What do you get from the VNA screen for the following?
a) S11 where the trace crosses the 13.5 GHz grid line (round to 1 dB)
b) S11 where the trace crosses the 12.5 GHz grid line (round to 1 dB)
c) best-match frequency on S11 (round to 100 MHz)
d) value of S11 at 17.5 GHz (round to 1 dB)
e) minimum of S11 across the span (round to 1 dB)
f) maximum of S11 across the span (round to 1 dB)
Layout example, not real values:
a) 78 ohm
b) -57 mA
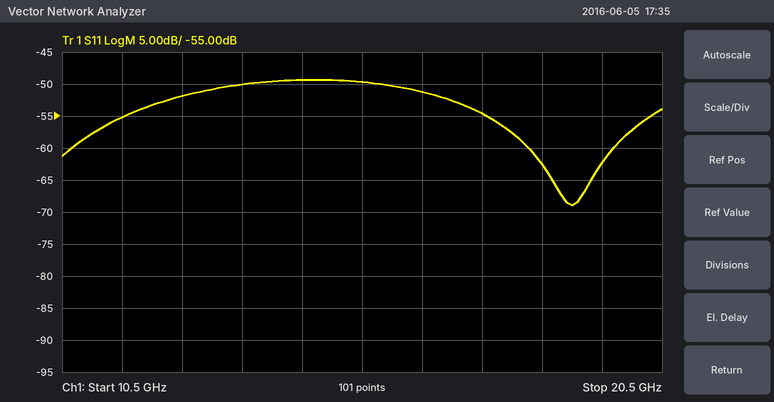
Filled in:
a) -50 dB
b) -52 dB
c) 19.0 GHz
d) -55 dB
e) -69 dB
f) -49 dB
